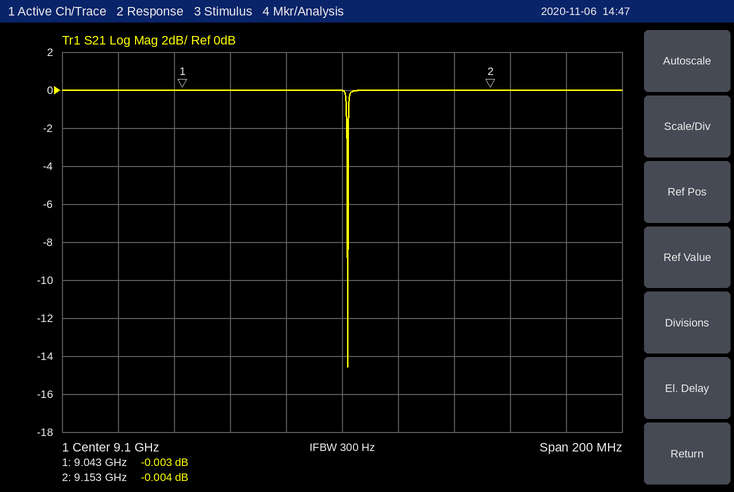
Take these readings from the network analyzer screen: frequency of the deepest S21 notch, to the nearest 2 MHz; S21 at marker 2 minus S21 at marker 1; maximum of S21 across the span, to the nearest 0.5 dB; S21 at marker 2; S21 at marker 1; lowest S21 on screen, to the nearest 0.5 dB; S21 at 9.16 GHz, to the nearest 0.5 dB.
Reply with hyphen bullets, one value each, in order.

- 9.102 GHz
- -0.001 dB
- 0.0 dB
- -0.004 dB
- -0.003 dB
- -14.5 dB
- 0.0 dB
